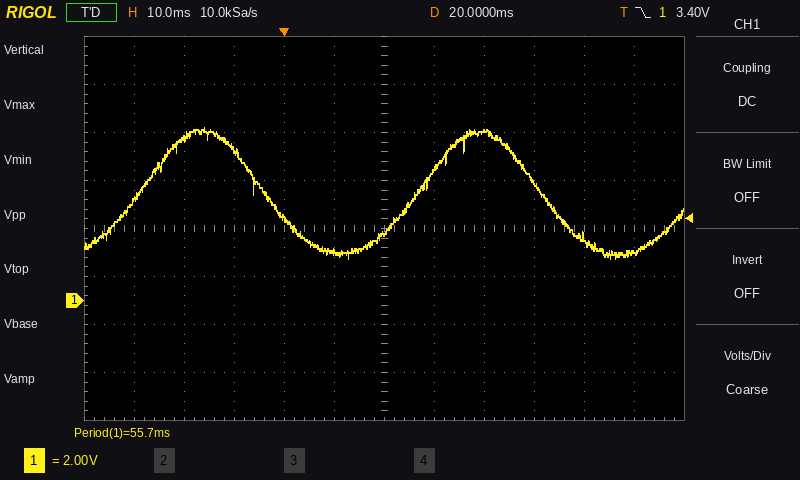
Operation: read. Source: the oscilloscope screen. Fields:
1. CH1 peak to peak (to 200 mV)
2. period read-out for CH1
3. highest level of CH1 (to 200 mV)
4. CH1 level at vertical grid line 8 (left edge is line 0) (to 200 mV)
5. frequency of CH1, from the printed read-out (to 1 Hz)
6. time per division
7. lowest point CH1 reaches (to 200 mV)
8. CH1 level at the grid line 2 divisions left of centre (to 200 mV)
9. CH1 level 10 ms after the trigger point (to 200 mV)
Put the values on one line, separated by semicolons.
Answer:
5.4 V; 55.7 ms; 7.2 V; 7.0 V; 18 Hz; 10 ms; 1.8 V; 3.4 V; 2.0 V
